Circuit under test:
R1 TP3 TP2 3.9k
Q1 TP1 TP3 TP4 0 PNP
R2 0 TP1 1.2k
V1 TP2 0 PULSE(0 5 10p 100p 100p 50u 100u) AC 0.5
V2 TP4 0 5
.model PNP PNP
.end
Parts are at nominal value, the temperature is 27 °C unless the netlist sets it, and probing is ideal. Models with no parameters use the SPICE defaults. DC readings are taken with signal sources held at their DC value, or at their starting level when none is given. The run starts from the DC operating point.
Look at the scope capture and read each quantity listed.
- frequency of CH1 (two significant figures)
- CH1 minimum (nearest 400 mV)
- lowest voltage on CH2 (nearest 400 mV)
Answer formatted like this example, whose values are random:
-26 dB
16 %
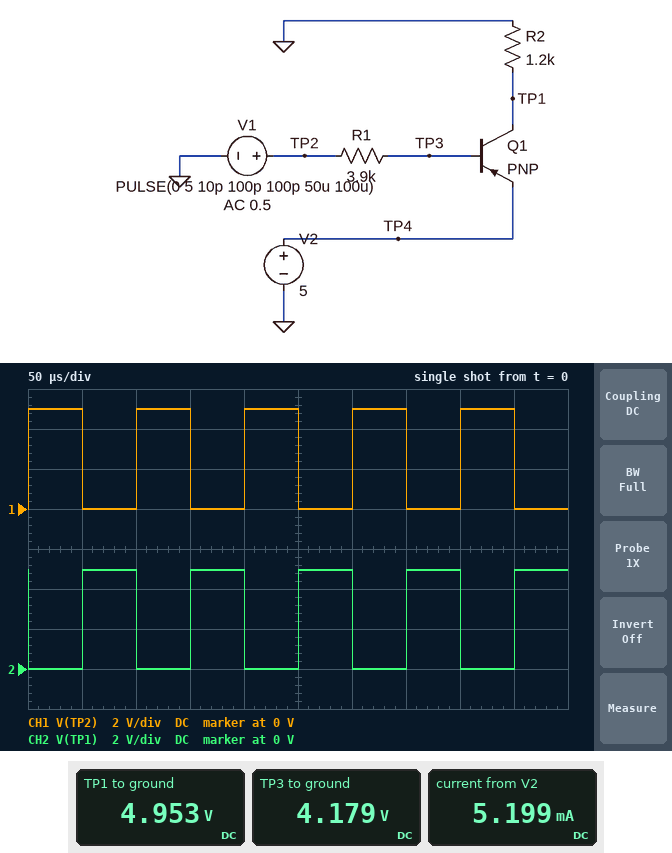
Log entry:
10 kHz
0 V
0 V
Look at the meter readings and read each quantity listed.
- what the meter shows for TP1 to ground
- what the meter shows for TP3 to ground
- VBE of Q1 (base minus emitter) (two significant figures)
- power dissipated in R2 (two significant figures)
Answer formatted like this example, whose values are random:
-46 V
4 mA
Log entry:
4.953 V
4.179 V
-820 mV
20 mW
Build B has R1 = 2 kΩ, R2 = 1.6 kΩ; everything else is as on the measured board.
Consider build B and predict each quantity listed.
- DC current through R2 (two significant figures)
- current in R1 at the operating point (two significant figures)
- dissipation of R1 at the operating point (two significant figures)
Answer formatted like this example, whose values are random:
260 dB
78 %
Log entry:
3.1 mA
2.1 mA
8.7 mW
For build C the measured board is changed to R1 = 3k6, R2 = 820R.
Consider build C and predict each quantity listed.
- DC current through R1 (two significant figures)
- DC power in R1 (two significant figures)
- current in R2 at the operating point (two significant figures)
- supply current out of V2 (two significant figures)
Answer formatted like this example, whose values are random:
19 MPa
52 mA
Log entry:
1.2 mA
4.8 mW
6.0 mA
7.2 mA
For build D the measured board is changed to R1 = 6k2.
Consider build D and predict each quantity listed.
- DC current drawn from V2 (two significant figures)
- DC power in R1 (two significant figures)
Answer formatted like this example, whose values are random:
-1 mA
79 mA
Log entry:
4.8 mA
2.8 mW
